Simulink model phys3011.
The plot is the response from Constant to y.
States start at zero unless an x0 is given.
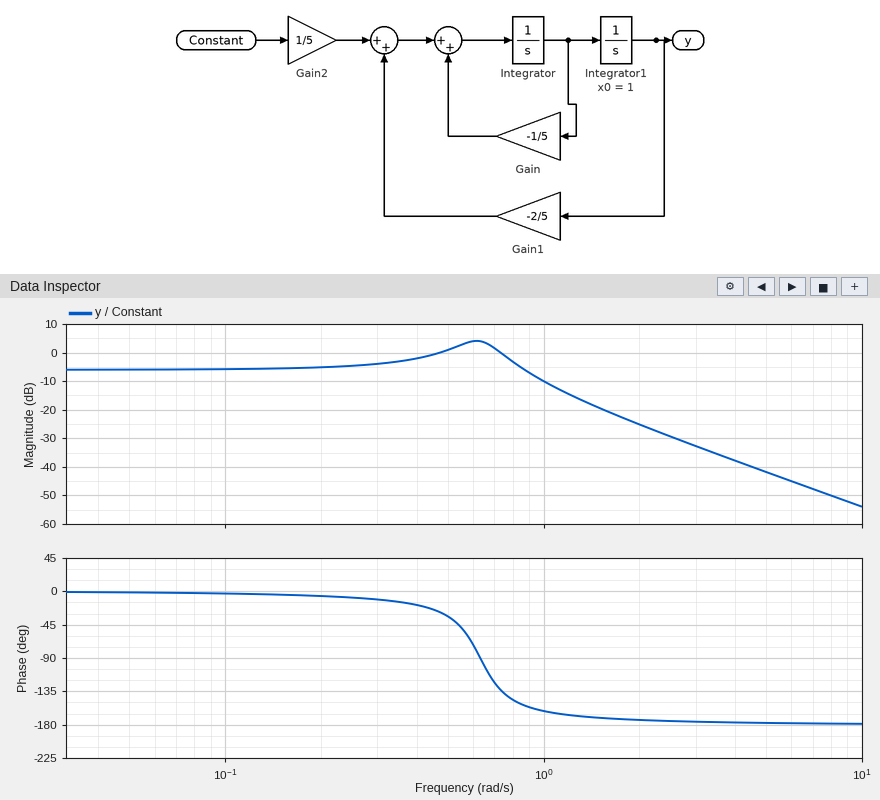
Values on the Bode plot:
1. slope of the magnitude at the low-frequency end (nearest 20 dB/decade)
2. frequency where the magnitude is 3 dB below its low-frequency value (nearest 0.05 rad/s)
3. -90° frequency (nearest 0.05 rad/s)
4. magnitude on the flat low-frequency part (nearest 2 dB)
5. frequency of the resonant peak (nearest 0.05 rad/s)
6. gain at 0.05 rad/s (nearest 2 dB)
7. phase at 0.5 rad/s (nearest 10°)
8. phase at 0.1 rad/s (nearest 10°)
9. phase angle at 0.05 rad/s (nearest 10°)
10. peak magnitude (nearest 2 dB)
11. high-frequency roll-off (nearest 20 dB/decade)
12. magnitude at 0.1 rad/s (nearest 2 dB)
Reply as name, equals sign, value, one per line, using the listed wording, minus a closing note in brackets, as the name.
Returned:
slope of the magnitude at the low-frequency end = 0 dB/decade
frequency where the magnitude is 3 dB below its low-frequency value = 0.95 rad/s
-90° frequency = 0.65 rad/s
magnitude on the flat low-frequency part = -6 dB
frequency of the resonant peak = 0.60 rad/s
gain at 0.05 rad/s = -6 dB
phase at 0.5 rad/s = -30°
phase at 0.1 rad/s = 0°
phase angle at 0.05 rad/s = 0°
peak magnitude = 4 dB
high-frequency roll-off = -40 dB/decade
magnitude at 0.1 rad/s = -6 dB
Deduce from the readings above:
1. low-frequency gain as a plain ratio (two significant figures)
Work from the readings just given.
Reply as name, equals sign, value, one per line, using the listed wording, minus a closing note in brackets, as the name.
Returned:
low-frequency gain as a plain ratio = 0.50
